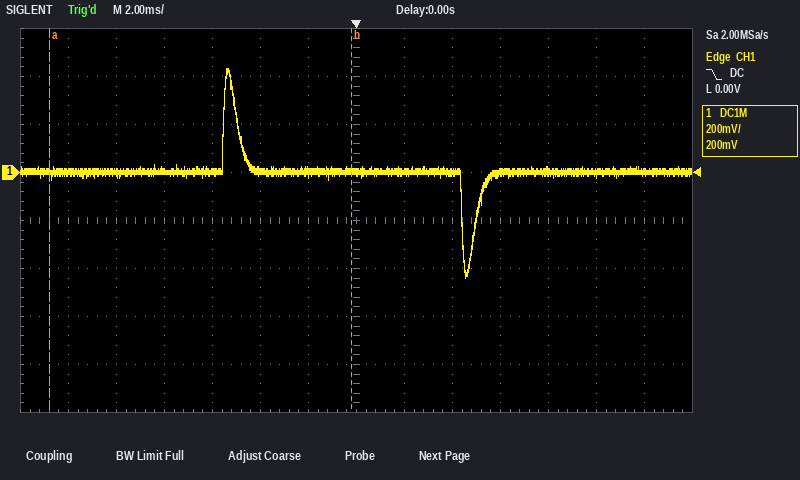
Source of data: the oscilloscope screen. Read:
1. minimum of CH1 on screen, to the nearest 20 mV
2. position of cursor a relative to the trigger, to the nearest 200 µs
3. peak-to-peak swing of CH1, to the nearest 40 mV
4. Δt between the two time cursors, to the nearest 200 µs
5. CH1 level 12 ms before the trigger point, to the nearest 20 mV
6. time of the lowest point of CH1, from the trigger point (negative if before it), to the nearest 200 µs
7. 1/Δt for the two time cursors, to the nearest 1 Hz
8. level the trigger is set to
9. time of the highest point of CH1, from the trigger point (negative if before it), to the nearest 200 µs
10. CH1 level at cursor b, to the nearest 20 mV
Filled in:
-440 mV
-12.8 ms
880 mV
12.6 ms
0 mV
+4.6 ms
79 Hz
0.00 V
-5.4 ms
0 mV
